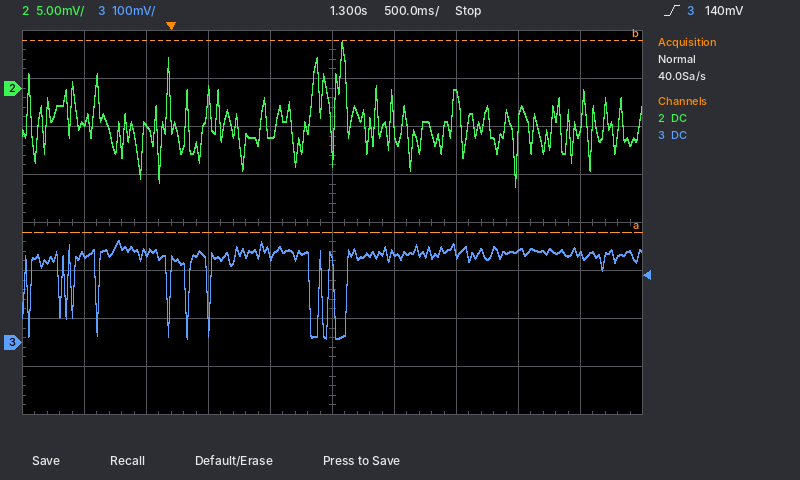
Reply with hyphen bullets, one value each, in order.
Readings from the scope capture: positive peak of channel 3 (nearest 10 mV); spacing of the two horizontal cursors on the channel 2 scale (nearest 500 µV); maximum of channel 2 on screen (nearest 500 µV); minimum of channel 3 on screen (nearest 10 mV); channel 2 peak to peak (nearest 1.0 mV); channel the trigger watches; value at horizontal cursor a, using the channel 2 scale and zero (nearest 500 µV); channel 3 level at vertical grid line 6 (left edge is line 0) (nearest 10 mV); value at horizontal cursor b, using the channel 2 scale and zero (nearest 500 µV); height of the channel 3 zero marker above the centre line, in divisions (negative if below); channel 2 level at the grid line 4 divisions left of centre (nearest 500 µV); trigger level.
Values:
- 210 mV
- 20.0 mV
- 5.0 mV
- 10 mV
- 15.0 mV
- channel 3
- -15.0 mV
- 190 mV
- 5.0 mV
- -2.5 div
- -3.5 mV
- 140 mV
